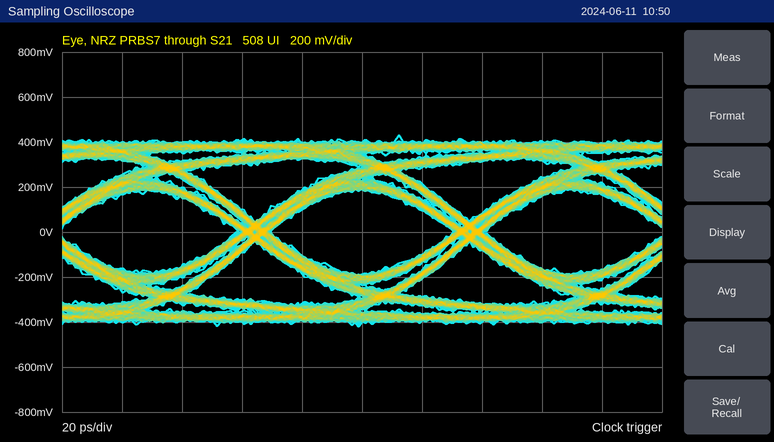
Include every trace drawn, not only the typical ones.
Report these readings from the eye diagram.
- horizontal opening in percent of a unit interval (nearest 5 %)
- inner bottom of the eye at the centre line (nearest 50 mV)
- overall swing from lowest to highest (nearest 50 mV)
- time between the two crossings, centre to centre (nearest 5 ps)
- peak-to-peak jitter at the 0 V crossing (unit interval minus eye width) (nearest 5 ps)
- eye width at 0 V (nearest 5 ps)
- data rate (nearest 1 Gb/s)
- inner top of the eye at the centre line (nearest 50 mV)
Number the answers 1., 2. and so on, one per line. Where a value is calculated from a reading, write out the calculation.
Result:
1. 60 ps / 70 ps ≈ 85.7 %, so 85 % to the nearest 5 %
2. -200 mV
3. 850 mV
4. 70 ps
5. 10 ps
6. 60 ps
7. 14 Gb/s
8. 200 mV
